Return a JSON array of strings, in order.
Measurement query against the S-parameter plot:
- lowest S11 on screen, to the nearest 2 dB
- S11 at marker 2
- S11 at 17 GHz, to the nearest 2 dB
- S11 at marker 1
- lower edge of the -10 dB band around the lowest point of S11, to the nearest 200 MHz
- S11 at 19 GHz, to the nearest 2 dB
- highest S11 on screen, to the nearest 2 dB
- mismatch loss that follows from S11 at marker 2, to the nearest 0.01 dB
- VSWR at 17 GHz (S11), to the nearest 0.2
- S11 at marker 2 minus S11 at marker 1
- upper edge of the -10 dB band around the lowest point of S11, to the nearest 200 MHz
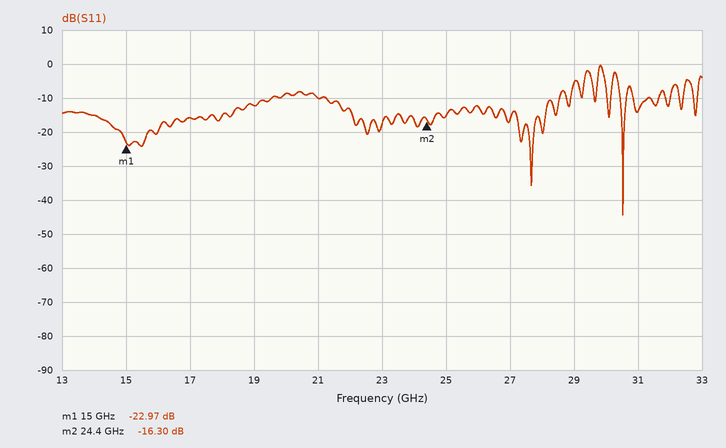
["-44 dB", "-16.30 dB", "-16 dB", "-22.97 dB", "30.4 GHz", "-12 dB", "0 dB", "0.10 dB", "1.4", "6.67 dB", "30.6 GHz"]
